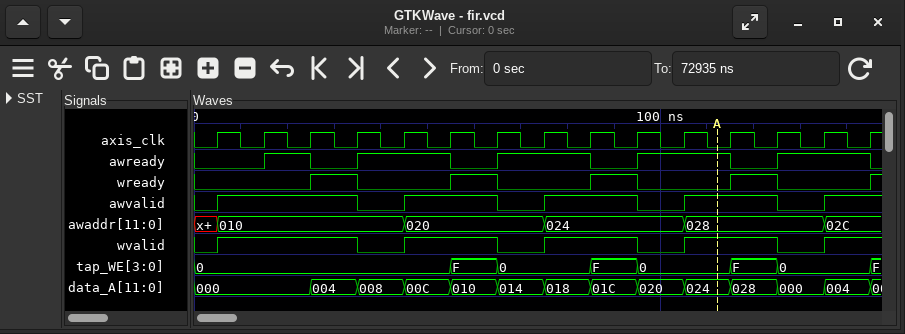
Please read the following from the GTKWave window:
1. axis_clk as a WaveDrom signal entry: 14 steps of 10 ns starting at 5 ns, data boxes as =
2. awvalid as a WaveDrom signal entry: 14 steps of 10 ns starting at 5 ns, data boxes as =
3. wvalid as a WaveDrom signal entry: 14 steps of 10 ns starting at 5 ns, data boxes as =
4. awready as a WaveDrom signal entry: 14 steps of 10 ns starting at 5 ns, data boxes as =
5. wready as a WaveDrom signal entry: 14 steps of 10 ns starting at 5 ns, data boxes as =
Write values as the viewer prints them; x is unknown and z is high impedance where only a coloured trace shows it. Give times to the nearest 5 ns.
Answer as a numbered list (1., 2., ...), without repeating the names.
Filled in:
1. {name: 'axis_clk', wave: 'p.............'}
2. {name: 'awvalid', wave: '1..01.01.01.01'}
3. {name: 'wvalid', wave: '1..01.01.01.01'}
4. {name: 'awready', wave: '0101.01.01.01.'}
5. {name: 'wready', wave: '0.10.10.10.10.'}
